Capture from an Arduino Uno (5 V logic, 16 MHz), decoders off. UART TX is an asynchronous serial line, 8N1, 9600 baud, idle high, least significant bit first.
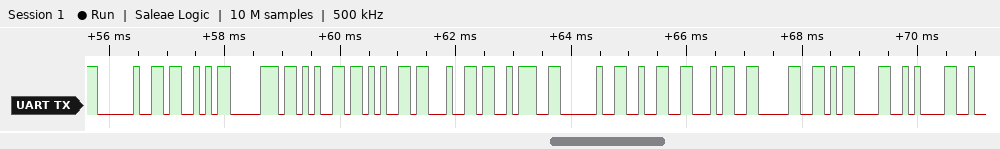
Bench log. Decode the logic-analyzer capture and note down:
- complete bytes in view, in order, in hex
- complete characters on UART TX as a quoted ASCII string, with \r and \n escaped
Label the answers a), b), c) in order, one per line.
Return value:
a) 20 53 70 65 65 64 3A 20 32 34 30 0D 0A
b) " Speed: 240\r\n"
